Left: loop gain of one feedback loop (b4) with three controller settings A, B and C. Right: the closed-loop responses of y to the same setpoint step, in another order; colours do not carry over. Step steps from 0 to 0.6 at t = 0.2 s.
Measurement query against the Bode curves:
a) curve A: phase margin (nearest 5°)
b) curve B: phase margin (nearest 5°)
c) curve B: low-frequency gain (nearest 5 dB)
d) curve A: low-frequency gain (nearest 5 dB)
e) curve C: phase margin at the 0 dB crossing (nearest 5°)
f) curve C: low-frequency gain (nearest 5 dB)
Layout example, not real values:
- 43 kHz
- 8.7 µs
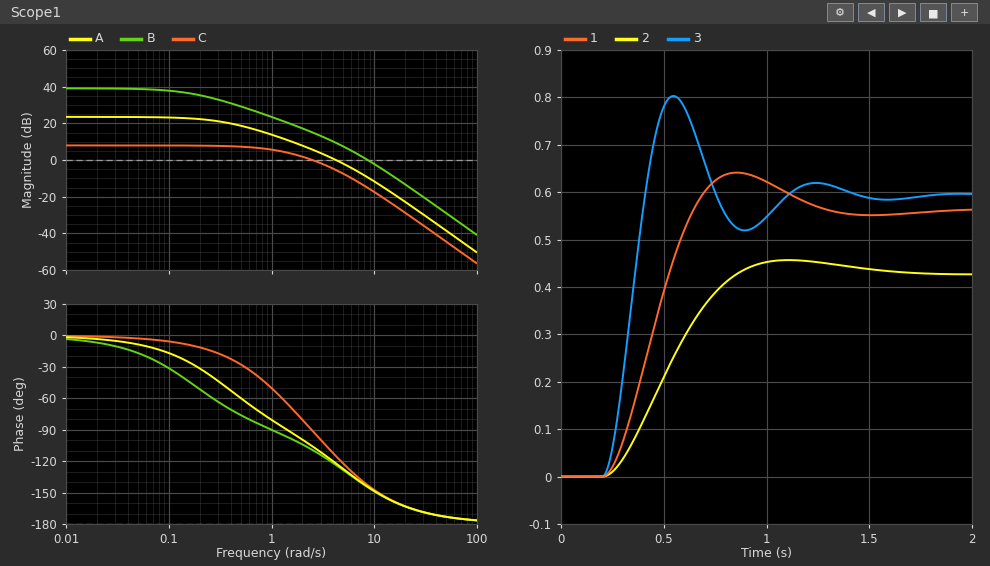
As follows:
- 60°
- 35°
- 40 dB
- 25 dB
- 90°
- 10 dB
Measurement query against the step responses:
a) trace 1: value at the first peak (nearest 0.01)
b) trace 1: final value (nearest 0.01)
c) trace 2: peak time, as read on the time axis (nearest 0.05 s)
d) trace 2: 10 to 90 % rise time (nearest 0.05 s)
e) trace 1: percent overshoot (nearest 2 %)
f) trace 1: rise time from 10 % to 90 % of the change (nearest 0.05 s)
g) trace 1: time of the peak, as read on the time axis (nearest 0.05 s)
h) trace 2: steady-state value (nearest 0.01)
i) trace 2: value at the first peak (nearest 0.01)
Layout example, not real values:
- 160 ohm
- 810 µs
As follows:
- 0.64
- 0.56
- 1.10 s
- 0.45 s
- 14 %
- 0.30 s
- 0.85 s
- 0.43
- 0.46
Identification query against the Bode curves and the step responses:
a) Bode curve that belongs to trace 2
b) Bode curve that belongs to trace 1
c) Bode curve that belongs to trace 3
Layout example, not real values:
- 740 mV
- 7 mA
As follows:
- C
- A
- B
